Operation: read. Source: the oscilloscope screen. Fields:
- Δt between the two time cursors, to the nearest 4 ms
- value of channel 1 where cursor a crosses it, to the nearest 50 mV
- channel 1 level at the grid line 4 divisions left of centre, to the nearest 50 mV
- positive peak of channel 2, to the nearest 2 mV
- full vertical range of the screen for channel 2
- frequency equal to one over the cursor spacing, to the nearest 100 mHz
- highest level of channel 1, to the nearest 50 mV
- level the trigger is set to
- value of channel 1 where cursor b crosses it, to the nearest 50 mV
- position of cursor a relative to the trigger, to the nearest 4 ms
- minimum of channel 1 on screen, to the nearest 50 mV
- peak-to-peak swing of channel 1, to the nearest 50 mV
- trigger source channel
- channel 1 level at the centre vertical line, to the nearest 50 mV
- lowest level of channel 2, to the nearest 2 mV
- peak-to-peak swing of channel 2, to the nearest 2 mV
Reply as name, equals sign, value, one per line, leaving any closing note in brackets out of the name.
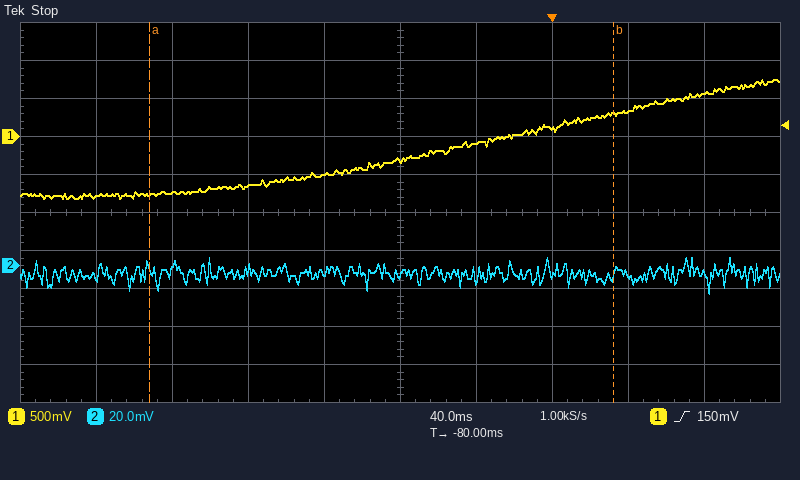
Δt between the two time cursors, to the nearest 4 ms = 244 ms
value of channel 1 where cursor a crosses it, to the nearest 50 mV = -750 mV
channel 1 level at the grid line 4 divisions left of centre, to the nearest 50 mV = -800 mV
positive peak of channel 2, to the nearest 2 mV = 4 mV
full vertical range of the screen for channel 2 = 200 mV
frequency equal to one over the cursor spacing, to the nearest 100 mHz = 4.1 Hz
highest level of channel 1, to the nearest 50 mV = 750 mV
level the trigger is set to = 150 mV
value of channel 1 where cursor b crosses it, to the nearest 50 mV = 300 mV
position of cursor a relative to the trigger, to the nearest 4 ms = -212 ms
minimum of channel 1 on screen, to the nearest 50 mV = -800 mV
peak-to-peak swing of channel 1, to the nearest 50 mV = 1.55 V
trigger source channel = channel 1
channel 1 level at the centre vertical line, to the nearest 50 mV = -300 mV
lowest level of channel 2, to the nearest 2 mV = -14 mV
peak-to-peak swing of channel 2, to the nearest 2 mV = 18 mV
